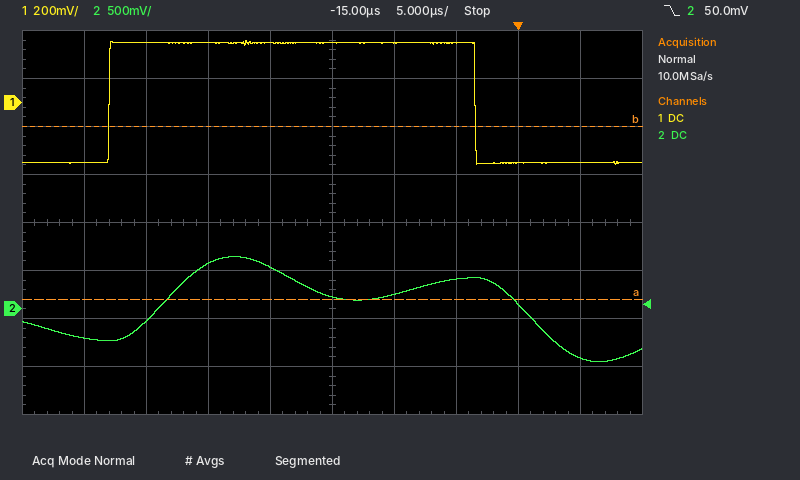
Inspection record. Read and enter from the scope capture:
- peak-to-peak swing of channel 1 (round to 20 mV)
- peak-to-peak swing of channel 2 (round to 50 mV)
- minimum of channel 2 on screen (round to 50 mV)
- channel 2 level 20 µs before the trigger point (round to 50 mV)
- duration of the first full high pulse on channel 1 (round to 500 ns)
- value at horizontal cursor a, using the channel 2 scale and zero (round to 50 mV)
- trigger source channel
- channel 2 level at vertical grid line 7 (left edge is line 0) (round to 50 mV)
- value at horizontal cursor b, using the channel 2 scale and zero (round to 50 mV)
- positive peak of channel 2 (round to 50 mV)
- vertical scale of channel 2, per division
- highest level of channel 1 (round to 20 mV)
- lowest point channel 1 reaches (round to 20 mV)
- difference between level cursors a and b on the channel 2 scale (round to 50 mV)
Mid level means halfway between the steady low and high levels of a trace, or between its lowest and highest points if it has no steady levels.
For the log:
520 mV
1.10 V
-550 mV
450 mV
29.5 µs
100 mV
channel 2
300 mV
1.90 V
550 mV
500 mV
260 mV
-260 mV
1.80 V
